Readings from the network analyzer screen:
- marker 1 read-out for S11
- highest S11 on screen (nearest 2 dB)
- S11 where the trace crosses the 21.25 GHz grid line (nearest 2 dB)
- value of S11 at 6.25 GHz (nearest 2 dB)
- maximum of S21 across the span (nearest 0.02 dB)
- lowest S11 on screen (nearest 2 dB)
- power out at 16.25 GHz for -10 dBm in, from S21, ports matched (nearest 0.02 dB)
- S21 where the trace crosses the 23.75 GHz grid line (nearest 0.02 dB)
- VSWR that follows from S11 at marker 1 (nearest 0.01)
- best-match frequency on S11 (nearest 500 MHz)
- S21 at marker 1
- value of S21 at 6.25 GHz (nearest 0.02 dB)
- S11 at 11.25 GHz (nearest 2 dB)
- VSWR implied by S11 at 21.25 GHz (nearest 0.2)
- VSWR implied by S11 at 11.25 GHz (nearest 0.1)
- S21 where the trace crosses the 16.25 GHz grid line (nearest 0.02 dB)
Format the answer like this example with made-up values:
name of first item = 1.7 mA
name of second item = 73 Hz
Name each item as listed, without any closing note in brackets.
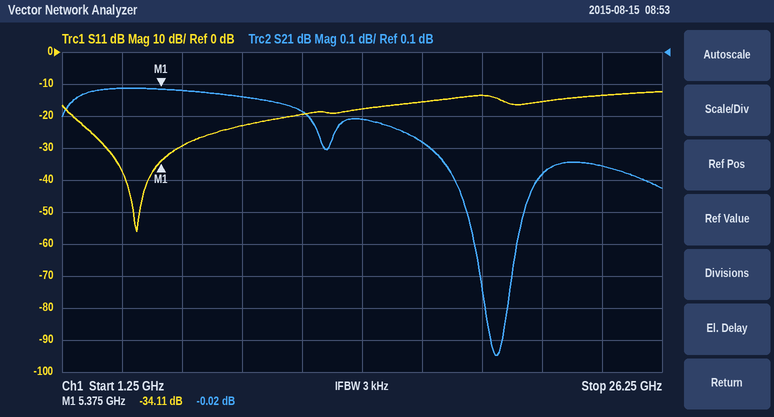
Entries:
marker 1 read-out for S11 = -34.11 dB
highest S11 on screen = -12 dB
S11 where the trace crosses the 21.25 GHz grid line = -16 dB
value of S11 at 6.25 GHz = -30 dB
maximum of S21 across the span = -0.02 dB
lowest S11 on screen = -56 dB
power out at 16.25 GHz for -10 dBm in, from S21, ports matched = -10.18 dBm
S21 where the trace crosses the 23.75 GHz grid line = -0.26 dB
VSWR that follows from S11 at marker 1 = 1.04
best-match frequency on S11 = 4.5 GHz
S21 at marker 1 = -0.02 dB
value of S21 at 6.25 GHz = -0.02 dB
S11 at 11.25 GHz = -20 dB
VSWR implied by S11 at 21.25 GHz = 1.4
VSWR implied by S11 at 11.25 GHz = 1.2
S21 where the trace crosses the 16.25 GHz grid line = -0.18 dB
